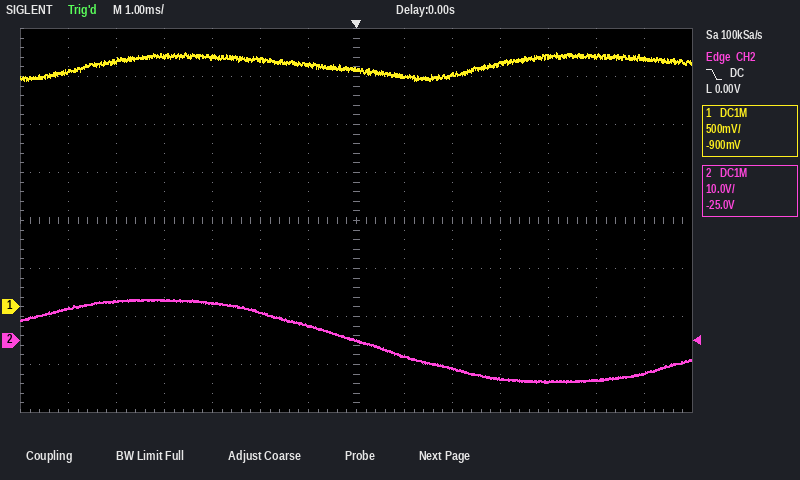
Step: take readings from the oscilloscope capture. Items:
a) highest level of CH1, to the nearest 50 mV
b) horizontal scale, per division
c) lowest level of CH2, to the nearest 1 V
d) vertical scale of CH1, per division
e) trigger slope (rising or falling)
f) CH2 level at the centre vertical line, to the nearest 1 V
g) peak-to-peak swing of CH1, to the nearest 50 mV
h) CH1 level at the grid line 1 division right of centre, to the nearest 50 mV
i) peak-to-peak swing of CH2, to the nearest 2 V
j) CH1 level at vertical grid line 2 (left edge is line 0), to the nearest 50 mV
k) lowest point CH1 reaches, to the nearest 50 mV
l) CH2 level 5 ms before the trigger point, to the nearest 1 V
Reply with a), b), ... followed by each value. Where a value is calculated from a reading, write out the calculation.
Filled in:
a) 2.65 V
b) 1 ms
c) -9 V
d) 500 mV
e) falling
f) 0 V
g) 2.65 V − (2.35 V) = 300 mV
h) 2.40 V
i) 18 V
j) 2.55 V
k) 2.35 V
l) 8 V
